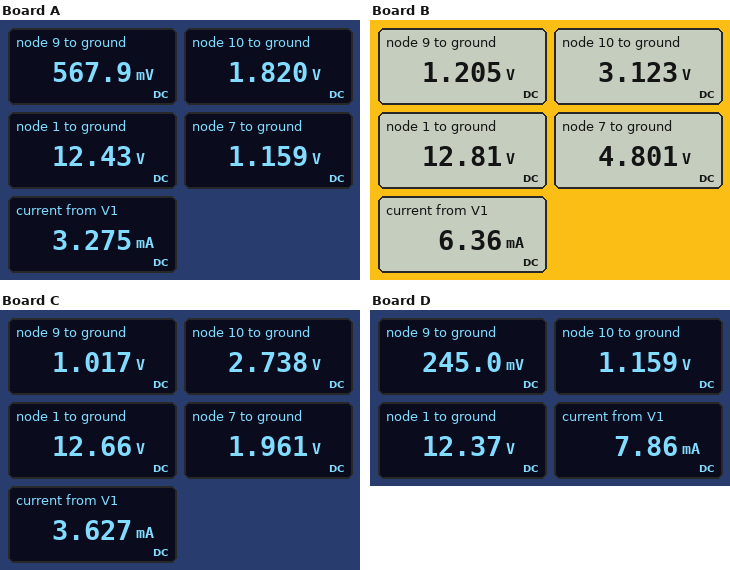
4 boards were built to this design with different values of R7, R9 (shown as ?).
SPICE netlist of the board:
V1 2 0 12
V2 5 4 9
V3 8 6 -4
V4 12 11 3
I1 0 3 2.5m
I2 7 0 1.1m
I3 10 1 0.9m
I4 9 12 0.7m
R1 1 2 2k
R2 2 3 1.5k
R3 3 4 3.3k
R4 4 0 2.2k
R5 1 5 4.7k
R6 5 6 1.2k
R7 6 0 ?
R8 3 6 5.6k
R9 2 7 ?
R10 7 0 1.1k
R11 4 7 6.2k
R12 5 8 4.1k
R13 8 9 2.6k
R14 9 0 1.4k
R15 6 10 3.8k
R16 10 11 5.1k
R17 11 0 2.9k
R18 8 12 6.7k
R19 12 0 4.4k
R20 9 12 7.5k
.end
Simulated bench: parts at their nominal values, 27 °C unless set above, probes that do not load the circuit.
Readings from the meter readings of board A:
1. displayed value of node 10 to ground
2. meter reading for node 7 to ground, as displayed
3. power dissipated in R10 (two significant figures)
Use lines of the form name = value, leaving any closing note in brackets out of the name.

displayed value of node 10 to ground = 1.820 V
meter reading for node 7 to ground, as displayed = 1.159 V
power dissipated in R10 = 1.2 mW
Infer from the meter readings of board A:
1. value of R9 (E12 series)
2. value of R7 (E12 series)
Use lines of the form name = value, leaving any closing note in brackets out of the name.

value of R9 = 4.7 kΩ
value of R7 = 2.7 kΩ
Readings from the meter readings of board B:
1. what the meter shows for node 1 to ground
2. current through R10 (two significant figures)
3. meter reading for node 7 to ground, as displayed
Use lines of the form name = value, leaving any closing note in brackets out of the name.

what the meter shows for node 1 to ground = 12.81 V
current through R10 = 4.4 mA
meter reading for node 7 to ground, as displayed = 4.801 V
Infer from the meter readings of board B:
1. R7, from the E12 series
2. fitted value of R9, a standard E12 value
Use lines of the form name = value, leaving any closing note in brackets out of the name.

R7, from the E12 series = 10 kΩ
fitted value of R9, a standard E12 value = 1.2 kΩ
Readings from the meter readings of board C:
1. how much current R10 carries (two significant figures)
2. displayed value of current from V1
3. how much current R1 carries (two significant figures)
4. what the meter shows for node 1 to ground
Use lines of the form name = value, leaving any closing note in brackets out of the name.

how much current R10 carries = 1.8 mA
displayed value of current from V1 = 3.627 mA
how much current R1 carries = 330 µA
what the meter shows for node 1 to ground = 12.66 V
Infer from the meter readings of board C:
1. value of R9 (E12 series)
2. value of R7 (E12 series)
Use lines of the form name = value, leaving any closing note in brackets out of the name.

value of R9 = 3.3 kΩ
value of R7 = 6.8 kΩ
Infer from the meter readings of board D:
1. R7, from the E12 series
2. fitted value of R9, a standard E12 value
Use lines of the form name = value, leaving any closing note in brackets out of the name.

R7, from the E12 series = 1.5 kΩ
fitted value of R9, a standard E12 value = 1 kΩ
